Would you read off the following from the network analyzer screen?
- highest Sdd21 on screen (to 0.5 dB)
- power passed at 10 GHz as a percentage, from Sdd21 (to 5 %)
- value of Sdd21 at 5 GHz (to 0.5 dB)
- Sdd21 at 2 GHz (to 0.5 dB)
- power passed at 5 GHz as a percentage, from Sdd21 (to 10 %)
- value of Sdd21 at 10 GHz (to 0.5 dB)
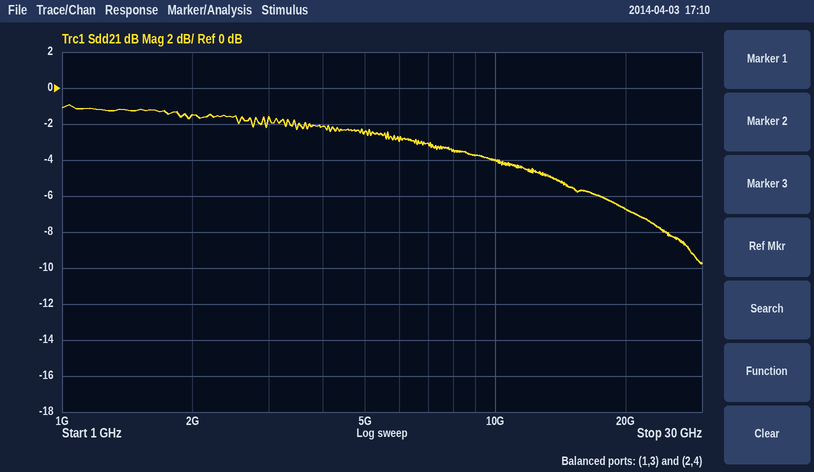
-1.0 dB
40 %
-2.5 dB
-1.5 dB
60 %
-4.0 dB
